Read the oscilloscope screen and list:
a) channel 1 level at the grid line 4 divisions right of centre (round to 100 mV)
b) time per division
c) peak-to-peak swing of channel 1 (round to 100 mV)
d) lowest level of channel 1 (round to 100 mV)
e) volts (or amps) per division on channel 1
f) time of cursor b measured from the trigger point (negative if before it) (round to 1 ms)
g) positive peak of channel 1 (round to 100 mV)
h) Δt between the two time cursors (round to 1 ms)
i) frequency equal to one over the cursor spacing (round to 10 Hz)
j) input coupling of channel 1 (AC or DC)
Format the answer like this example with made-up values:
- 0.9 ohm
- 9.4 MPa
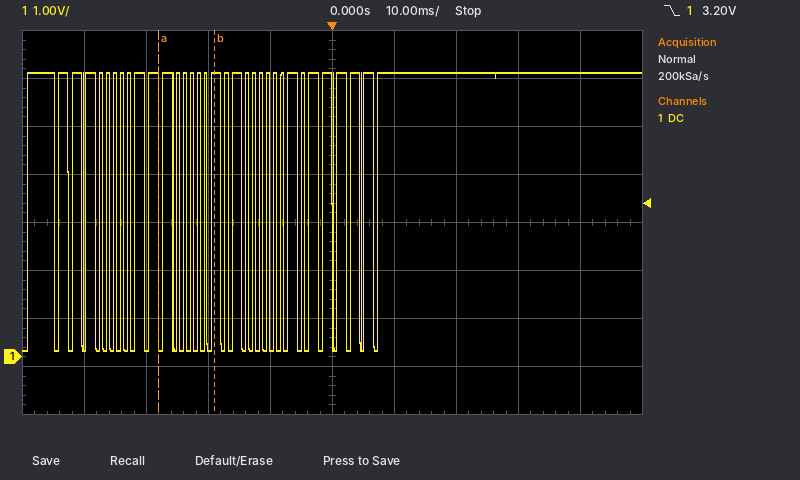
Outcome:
- 5.9 V
- 10 ms
- 5.8 V
- 100 mV
- 1 V
- -19 ms
- 5.9 V
- 9 ms
- 110 Hz
- DC
